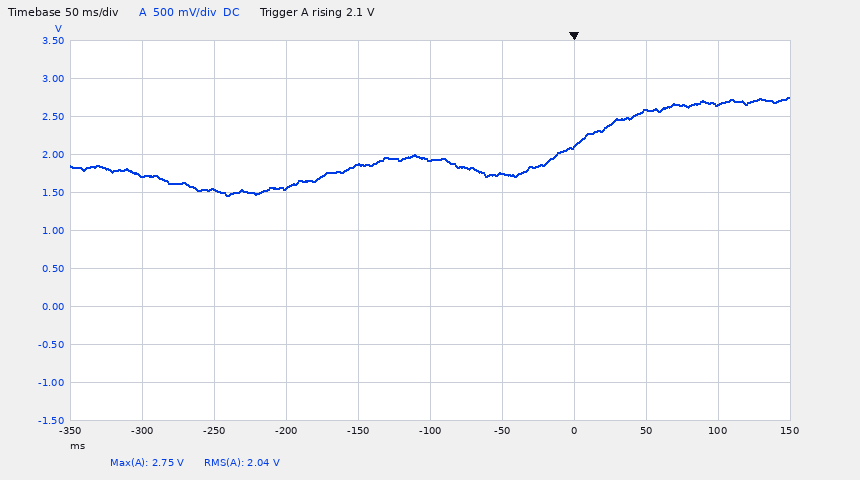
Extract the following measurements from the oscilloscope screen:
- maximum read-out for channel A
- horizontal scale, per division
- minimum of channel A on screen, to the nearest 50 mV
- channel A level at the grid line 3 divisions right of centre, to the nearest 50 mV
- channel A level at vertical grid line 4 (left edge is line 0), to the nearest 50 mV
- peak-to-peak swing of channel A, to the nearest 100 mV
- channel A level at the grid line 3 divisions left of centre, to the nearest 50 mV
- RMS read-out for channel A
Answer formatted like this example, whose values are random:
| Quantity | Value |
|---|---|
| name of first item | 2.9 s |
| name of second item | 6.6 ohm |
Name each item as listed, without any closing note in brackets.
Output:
| Quantity | Value |
|---|---|
| maximum read-out for channel A | 2.75 V |
| horizontal scale, per division | 50 ms |
| minimum of channel A on screen, to the nearest 50 mV | 1.45 V |
| channel A level at the grid line 3 divisions right of centre, to the nearest 50 mV | 2.60 V |
| channel A level at vertical grid line 4 (left edge is line 0), to the nearest 50 mV | 1.85 V |
| peak-to-peak swing of channel A, to the nearest 100 mV | 1.30 V |
| channel A level at the grid line 3 divisions left of centre, to the nearest 50 mV | 1.55 V |
| RMS read-out for channel A | 2.04 V |
